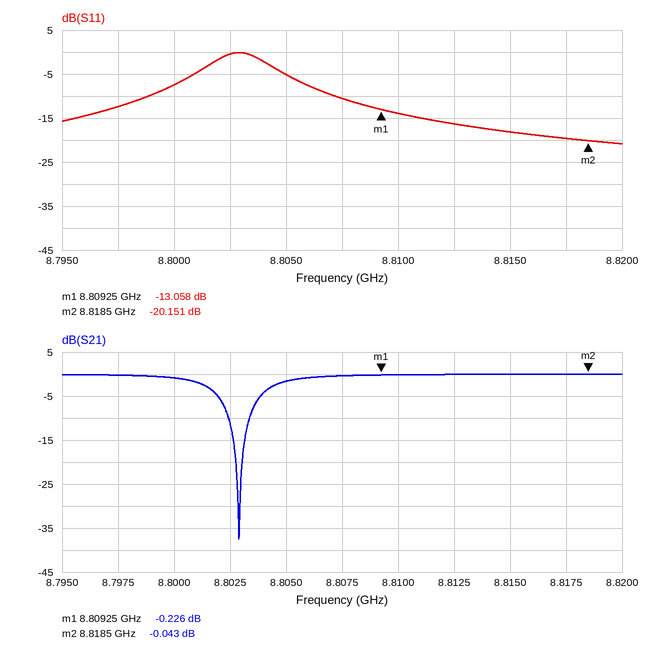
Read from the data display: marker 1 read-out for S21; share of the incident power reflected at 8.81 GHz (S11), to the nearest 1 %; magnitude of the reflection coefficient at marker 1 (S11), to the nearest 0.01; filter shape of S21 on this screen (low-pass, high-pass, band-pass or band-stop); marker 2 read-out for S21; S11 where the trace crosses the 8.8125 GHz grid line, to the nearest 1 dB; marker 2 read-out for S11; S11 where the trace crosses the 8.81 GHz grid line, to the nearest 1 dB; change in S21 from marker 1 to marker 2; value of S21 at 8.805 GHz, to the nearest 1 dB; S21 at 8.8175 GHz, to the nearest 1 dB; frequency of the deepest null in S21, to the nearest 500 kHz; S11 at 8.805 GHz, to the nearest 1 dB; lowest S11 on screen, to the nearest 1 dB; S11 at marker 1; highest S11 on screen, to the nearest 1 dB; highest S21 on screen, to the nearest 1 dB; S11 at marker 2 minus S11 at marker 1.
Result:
-0.226 dB
4 %
0.22
band-stop
-0.043 dB
-16 dB
-20.151 dB
-14 dB
0.183 dB
-2 dB
0 dB
8.8030 GHz
-5 dB
-21 dB
-13.058 dB
0 dB
0 dB
-7.093 dB
